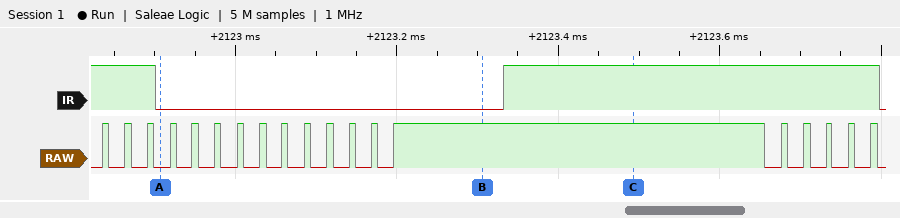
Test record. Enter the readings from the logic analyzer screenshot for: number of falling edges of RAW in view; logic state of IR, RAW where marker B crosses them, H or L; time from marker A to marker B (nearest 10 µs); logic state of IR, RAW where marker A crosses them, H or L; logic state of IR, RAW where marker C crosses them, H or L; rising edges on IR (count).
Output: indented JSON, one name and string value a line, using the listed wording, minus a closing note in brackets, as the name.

{
  "number of falling edges of RAW in view": "19",
  "logic state of IR, RAW where marker B crosses them, H or L": "IR=L, RAW=H",
  "time from marker A to marker B": "400 µs",
  "logic state of IR, RAW where marker A crosses them, H or L": "IR=L, RAW=L",
  "logic state of IR, RAW where marker C crosses them, H or L": "IR=H, RAW=H",
  "rising edges on IR": "1"
}
